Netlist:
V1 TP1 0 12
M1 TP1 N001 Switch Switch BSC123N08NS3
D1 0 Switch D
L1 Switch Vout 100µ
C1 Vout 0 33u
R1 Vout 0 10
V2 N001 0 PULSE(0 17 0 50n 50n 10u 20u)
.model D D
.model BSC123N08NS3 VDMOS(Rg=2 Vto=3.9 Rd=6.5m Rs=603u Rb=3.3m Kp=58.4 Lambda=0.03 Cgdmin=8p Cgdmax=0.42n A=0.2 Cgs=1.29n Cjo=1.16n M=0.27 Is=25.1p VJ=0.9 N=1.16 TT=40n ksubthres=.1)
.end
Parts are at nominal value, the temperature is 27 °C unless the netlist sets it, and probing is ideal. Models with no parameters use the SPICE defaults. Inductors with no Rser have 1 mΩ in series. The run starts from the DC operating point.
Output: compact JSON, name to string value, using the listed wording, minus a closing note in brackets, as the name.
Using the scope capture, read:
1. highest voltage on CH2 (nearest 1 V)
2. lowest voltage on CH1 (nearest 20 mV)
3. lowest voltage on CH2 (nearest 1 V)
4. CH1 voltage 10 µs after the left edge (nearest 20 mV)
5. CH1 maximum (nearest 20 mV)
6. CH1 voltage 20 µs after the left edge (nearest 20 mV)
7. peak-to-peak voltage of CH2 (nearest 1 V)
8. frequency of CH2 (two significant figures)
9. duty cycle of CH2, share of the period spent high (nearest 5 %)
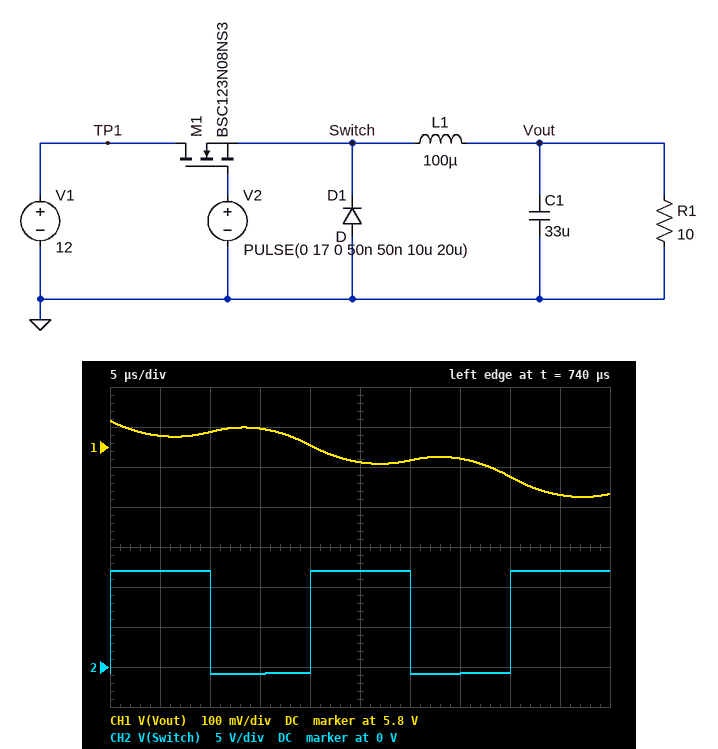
{"highest voltage on CH2": "12 V", "lowest voltage on CH1": "5.68 V", "lowest voltage on CH2": "-1 V", "CH1 voltage 10 µs after the left edge": "5.84 V", "CH1 maximum": "5.86 V", "CH1 voltage 20 µs after the left edge": "5.80 V", "peak-to-peak voltage of CH2": "13 V", "frequency of CH2": "50 kHz", "duty cycle of CH2, share of the period spent high": "50 %"}
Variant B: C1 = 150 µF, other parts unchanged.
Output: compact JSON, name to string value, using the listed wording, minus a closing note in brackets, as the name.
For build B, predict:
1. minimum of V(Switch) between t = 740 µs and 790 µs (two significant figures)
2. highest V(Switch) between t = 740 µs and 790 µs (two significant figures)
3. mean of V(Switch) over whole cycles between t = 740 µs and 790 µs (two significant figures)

{"minimum of V(Switch) between t = 740 µs and 790 µs": "-830 mV", "highest V(Switch) between t = 740 µs and 790 µs": "13 V", "mean of V(Switch) over whole cycles between t = 740 µs and 790 µs": "8.4 V"}
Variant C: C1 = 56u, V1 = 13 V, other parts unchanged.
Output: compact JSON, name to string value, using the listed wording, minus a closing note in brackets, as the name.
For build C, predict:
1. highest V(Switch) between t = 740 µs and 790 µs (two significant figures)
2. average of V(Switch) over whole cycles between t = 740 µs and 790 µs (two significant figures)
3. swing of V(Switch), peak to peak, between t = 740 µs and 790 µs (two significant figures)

{"highest V(Switch) between t = 740 µs and 790 µs": "13 V", "average of V(Switch) over whole cycles between t = 740 µs and 790 µs": "6.1 V", "swing of V(Switch), peak to peak, between t = 740 µs and 790 µs": "14 V"}
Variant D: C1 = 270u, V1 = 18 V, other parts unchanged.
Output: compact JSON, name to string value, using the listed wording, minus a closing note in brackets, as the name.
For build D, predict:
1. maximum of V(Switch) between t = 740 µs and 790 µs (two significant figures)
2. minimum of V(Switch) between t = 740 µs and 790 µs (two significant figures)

{"maximum of V(Switch) between t = 740 µs and 790 µs": "19 V", "minimum of V(Switch) between t = 740 µs and 790 µs": "-830 mV"}
